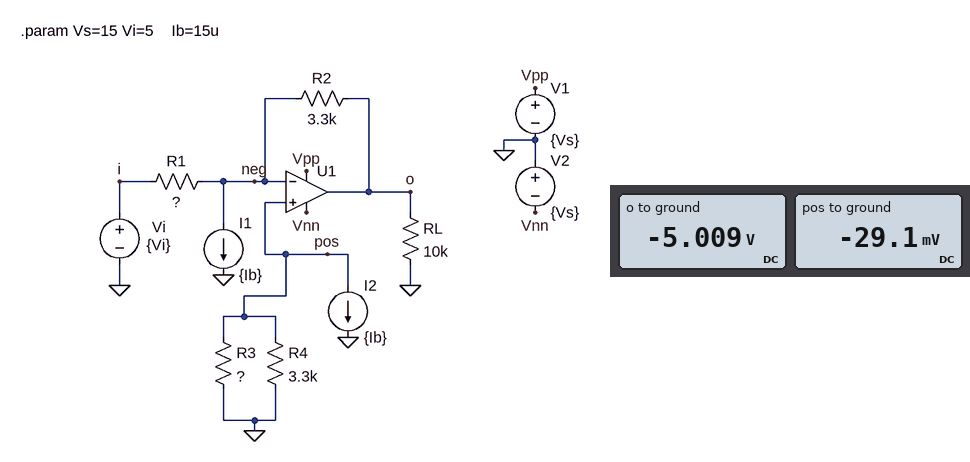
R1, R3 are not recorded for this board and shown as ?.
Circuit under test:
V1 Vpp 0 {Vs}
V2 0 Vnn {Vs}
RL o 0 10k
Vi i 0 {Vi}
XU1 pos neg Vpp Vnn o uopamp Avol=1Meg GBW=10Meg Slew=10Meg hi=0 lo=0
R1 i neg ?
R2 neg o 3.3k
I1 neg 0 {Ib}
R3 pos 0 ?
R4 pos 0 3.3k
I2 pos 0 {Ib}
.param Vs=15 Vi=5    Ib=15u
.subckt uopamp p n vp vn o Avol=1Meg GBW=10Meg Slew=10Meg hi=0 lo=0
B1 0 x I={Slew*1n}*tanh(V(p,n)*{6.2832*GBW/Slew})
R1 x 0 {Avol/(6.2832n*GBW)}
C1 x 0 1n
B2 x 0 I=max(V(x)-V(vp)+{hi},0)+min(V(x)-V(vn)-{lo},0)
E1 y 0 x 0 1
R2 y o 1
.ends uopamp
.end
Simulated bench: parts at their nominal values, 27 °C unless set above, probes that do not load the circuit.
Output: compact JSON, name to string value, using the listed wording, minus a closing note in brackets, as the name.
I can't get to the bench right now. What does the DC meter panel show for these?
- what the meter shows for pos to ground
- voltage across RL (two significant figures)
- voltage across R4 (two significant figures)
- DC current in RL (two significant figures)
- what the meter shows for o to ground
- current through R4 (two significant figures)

{"what the meter shows for pos to ground": "-29.1 mV", "voltage across RL": "5.0 V", "voltage across R4": "29 mV", "DC current in RL": "500 µA", "what the meter shows for o to ground": "-5.009 V", "current through R4": "8.8 µA"}
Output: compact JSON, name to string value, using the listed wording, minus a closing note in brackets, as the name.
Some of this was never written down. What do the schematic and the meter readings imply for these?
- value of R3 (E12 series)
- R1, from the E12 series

{"value of R3": "4.7 kΩ", "R1, from the E12 series": "3.3 kΩ"}
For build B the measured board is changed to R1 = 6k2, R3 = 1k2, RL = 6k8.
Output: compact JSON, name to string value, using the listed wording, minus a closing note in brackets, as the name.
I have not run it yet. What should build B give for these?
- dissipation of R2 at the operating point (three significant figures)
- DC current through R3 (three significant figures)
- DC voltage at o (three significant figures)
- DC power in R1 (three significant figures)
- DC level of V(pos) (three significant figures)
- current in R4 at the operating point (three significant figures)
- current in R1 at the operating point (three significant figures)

{"dissipation of R2 at the operating point": "2.08 mW", "DC current through R3": "11.0 µA", "DC voltage at o": "-2.63 V", "DC power in R1": "4.05 mW", "DC level of V(pos)": "-13.2 mV", "current in R4 at the operating point": "4.00 µA", "current in R1 at the operating point": "809 µA"}
